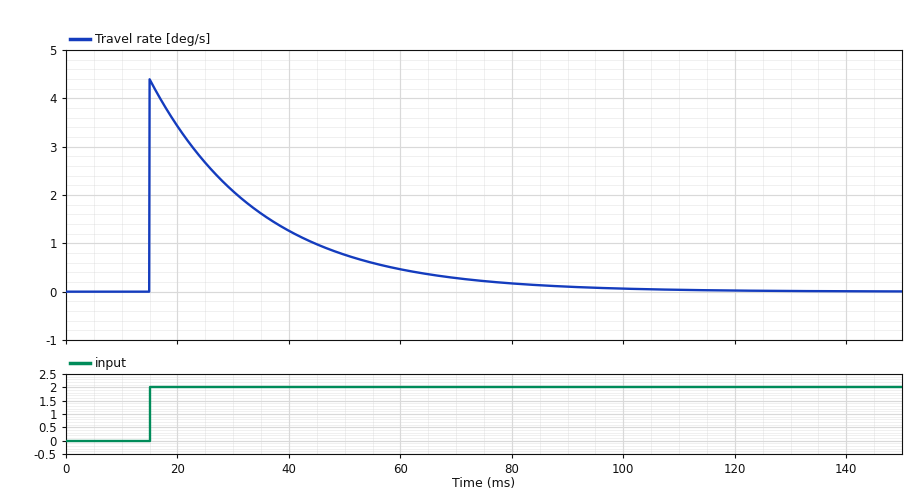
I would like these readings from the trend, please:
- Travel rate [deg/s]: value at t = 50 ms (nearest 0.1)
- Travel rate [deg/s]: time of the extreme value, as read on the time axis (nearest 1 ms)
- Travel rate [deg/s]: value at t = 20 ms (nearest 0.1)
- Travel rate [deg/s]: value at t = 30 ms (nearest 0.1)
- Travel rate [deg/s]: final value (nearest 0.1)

0.8
15 ms
3.4
2.1
0.0
